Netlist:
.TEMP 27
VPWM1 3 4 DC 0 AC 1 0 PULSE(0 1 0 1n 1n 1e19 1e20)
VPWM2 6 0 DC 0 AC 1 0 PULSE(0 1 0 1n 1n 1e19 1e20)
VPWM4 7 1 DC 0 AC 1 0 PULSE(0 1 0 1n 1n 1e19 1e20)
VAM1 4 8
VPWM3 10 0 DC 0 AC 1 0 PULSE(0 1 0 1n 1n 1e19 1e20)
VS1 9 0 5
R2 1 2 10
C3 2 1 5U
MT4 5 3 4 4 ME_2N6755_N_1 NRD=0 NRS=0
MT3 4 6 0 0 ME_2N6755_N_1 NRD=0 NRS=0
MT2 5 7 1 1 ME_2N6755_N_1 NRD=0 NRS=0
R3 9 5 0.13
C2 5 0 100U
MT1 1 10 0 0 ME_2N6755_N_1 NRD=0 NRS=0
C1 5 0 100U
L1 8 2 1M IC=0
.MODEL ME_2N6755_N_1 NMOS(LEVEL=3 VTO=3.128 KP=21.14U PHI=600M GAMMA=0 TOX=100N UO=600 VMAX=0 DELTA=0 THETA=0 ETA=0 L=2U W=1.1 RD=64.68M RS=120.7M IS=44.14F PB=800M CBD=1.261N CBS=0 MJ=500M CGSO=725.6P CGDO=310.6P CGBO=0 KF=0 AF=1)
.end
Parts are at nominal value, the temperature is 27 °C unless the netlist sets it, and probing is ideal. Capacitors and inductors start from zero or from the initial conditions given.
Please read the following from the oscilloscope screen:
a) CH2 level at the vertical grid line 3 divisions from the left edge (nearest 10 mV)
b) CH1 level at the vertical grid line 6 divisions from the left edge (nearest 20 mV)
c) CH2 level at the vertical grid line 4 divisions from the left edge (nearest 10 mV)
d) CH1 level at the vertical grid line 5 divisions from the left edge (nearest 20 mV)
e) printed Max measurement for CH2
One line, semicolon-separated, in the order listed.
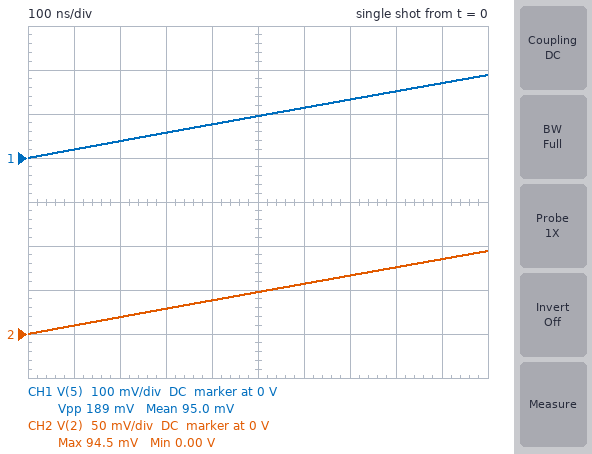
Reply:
30 mV; 120 mV; 40 mV; 100 mV; 94.5 mV
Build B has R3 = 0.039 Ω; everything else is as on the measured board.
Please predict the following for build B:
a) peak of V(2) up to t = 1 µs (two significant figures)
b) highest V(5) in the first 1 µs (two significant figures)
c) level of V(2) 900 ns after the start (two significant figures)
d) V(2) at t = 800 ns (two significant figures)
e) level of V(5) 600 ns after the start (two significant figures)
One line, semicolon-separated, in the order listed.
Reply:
300 mV; 600 mV; 270 mV; 240 mV; 370 mV
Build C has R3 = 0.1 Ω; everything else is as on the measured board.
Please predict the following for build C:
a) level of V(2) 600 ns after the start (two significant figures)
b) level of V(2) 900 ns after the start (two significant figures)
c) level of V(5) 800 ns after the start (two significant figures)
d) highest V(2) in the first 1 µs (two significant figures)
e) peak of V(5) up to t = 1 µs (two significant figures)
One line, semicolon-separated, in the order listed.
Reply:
74 mV; 110 mV; 200 mV; 120 mV; 240 mV
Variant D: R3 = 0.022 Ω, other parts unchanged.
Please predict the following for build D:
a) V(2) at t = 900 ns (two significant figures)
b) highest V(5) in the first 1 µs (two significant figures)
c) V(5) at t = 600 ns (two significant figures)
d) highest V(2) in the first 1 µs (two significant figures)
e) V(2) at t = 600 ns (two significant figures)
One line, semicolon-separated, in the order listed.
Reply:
460 mV; 1.0 V; 640 mV; 510 mV; 320 mV
